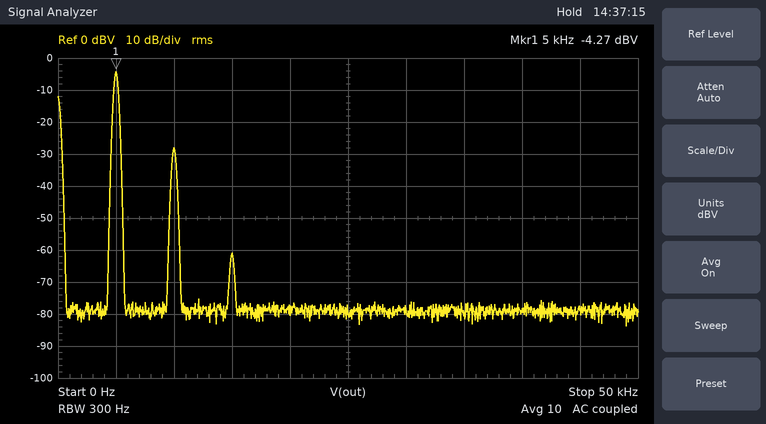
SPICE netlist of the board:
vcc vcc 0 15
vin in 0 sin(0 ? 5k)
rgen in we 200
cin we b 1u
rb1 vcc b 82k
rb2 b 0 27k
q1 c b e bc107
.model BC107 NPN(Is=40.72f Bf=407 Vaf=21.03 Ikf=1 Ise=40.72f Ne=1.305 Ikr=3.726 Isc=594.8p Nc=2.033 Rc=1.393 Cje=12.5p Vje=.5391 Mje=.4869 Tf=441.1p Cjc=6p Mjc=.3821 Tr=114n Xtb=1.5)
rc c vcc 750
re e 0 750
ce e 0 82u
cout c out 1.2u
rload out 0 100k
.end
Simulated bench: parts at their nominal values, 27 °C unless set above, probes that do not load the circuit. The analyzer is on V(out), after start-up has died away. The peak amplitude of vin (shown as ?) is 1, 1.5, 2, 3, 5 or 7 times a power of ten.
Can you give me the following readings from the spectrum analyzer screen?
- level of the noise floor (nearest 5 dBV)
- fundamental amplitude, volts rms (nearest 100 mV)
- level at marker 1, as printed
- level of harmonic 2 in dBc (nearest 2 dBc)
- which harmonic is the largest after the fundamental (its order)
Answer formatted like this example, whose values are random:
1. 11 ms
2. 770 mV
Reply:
1. -80 dBV
2. 600 mV
3. -4.27 dBV
4. -24 dBc
5. 2
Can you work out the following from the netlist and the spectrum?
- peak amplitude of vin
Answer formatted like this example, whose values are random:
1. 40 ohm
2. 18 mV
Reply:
1. 10 mV
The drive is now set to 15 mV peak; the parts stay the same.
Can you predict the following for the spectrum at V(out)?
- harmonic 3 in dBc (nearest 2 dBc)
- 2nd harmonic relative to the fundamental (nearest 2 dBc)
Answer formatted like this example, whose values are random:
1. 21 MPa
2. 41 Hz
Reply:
1. -50 dBc
2. -20 dBc
